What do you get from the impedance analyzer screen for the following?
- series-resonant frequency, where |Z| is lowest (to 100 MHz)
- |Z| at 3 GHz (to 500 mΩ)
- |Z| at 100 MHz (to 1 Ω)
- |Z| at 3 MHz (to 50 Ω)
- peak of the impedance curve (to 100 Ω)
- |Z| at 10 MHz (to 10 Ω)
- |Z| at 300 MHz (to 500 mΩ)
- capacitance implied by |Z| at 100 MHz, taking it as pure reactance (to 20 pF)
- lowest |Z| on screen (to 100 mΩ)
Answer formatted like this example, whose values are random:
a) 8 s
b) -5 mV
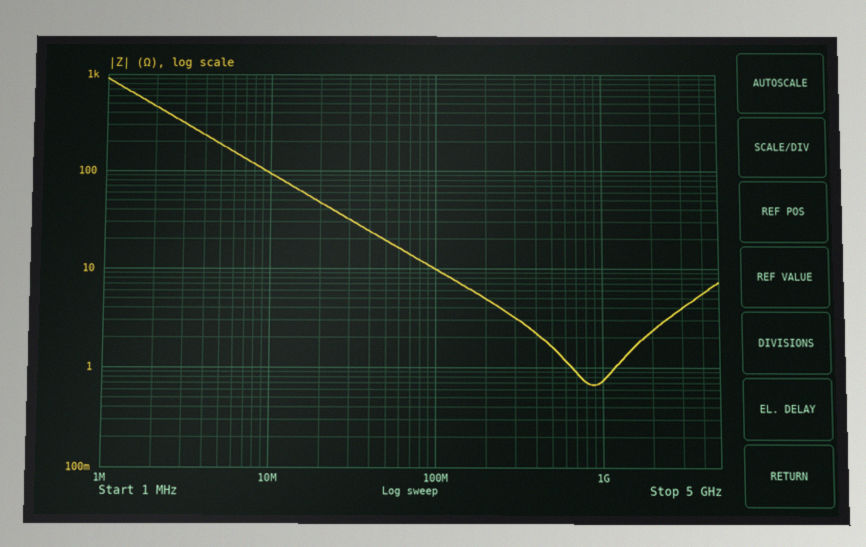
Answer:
a) 900 MHz
b) 4.0 Ω
c) 10 Ω
d) 300 Ω
e) 900 Ω
f) 90 Ω
g) 3.0 Ω
h) 160 pF
i) 700 mΩ
